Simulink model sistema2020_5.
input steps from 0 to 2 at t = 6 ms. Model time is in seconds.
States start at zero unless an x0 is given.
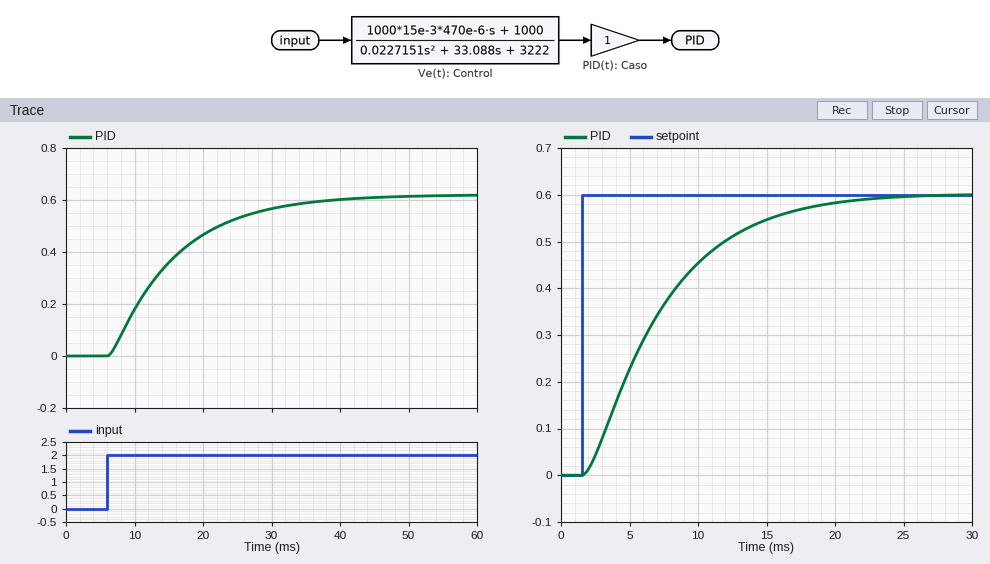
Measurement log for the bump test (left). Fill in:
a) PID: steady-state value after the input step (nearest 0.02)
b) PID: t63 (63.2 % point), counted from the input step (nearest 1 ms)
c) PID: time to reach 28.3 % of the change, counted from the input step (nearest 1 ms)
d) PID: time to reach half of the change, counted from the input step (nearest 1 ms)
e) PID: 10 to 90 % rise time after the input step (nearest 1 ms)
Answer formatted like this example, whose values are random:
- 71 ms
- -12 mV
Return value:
- 0.62
- 10 ms
- 4 ms
- 7 ms
- 21 ms
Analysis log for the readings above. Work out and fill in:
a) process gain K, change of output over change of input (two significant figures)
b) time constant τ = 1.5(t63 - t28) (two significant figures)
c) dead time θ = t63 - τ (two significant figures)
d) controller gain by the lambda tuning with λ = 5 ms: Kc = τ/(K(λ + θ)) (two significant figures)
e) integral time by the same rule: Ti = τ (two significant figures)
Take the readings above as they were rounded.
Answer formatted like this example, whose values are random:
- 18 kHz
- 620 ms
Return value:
- 0.31
- 9.0 ms
- 1.0 ms
- 4.8
- 9.0 ms
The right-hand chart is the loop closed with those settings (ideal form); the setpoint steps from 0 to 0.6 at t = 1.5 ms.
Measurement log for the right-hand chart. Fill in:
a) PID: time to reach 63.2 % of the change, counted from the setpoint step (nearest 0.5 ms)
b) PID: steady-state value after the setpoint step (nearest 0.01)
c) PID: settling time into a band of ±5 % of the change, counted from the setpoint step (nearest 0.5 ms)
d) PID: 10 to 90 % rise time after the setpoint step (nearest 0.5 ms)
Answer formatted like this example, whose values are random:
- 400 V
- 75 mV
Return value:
- 6.5 ms
- 0.60
- 16.0 ms
- 11.5 ms
